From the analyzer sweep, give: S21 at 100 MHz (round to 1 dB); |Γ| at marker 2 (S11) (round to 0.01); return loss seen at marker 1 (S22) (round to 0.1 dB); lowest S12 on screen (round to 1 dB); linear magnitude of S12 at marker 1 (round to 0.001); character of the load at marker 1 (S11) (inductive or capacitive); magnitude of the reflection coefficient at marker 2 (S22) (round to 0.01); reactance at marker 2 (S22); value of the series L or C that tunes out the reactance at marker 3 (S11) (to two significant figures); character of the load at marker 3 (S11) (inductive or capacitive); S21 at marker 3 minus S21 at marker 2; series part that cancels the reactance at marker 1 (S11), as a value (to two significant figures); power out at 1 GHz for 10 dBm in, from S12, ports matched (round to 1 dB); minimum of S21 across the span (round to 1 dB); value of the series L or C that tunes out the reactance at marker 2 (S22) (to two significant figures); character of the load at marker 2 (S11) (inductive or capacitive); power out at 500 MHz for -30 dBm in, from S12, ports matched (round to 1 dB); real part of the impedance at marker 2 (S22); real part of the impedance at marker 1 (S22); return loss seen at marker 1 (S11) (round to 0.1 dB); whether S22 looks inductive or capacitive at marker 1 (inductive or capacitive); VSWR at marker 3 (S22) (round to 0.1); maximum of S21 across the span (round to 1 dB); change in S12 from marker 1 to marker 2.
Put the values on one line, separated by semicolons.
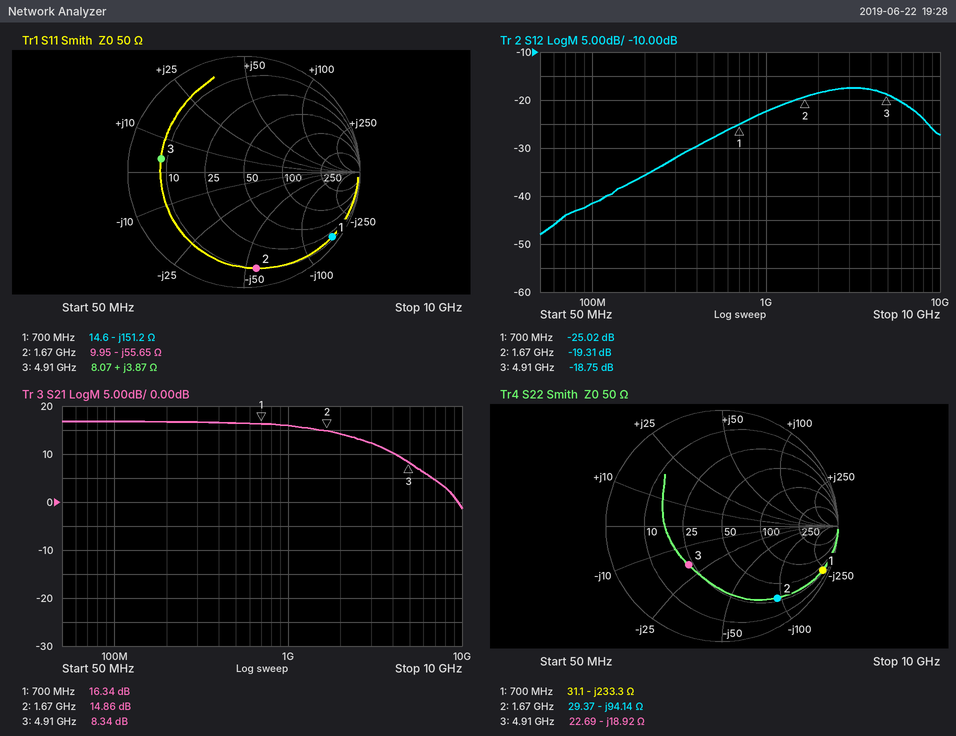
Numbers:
17 dB; 0.84; 0.5 dB; -48 dB; 0.056; capacitive; 0.78; -94.14 Ω; 8.4 pF; inductive; -6.52 dB; 34 nH; -12 dBm; -1 dB; 9.0 nH; capacitive; -58 dBm; 29.37 Ω; 31.1 Ω; 0.5 dB; capacitive; 2.6; 17 dB; 5.71 dB
